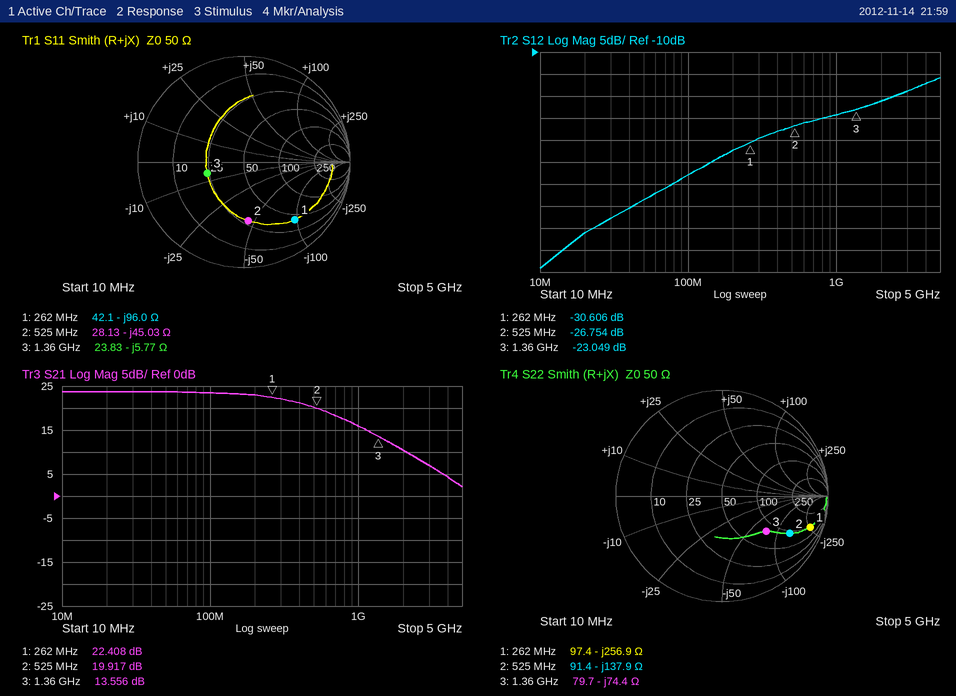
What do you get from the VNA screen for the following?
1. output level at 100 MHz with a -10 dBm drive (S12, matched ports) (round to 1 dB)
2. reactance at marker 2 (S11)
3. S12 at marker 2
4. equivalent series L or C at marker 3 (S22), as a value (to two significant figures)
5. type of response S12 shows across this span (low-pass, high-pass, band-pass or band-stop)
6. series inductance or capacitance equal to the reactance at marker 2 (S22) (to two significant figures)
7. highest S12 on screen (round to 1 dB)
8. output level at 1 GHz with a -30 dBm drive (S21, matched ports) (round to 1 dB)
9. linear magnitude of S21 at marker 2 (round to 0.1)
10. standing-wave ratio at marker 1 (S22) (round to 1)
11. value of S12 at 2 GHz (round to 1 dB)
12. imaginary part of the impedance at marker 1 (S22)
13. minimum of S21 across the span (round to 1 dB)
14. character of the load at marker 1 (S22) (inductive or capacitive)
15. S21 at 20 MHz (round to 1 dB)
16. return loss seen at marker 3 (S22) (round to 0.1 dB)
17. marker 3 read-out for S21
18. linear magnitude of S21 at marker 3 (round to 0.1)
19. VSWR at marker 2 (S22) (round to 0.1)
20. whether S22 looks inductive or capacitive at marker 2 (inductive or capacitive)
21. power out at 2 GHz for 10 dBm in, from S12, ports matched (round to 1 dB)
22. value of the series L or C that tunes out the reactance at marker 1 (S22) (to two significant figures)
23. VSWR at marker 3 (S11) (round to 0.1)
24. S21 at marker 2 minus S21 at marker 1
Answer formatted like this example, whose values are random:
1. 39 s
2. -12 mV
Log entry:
1. -48 dBm
2. -45.03 Ω
3. -26.754 dB
4. 1.6 pF
5. high-pass
6. 2.2 pF
7. -16 dB
8. -14 dBm
9. 9.9
10. 16
11. -21 dB
12. -256.9 Ω
13. 2 dB
14. capacitive
15. 24 dB
16. 5.4 dB
17. 13.556 dB
18. 4.8
19. 6.4
20. capacitive
21. -11 dBm
22. 160 nH
23. 2.1
24. -2.491 dB
